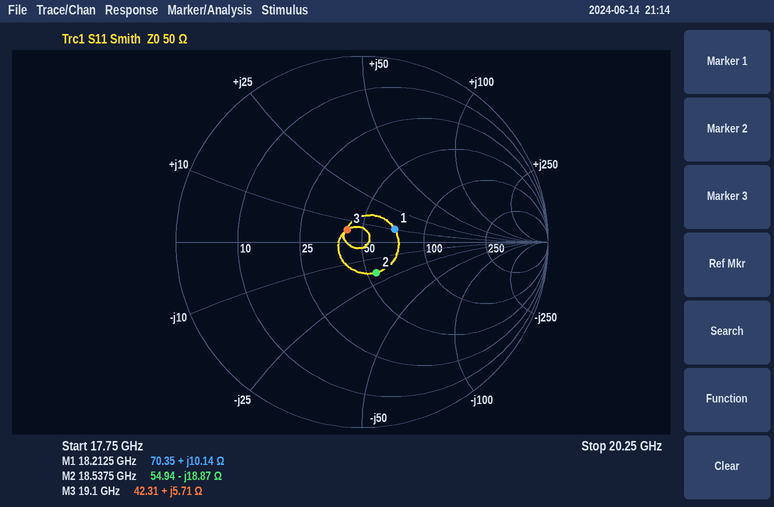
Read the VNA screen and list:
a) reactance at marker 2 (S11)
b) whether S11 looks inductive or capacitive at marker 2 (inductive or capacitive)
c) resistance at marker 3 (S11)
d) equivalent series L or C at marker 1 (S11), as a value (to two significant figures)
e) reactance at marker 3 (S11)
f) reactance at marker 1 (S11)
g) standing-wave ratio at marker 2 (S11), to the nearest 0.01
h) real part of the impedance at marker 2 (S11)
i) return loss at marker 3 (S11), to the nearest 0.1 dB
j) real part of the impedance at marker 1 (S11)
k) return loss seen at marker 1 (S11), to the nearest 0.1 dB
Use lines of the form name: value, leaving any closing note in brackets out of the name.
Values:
reactance at marker 2: -18.87 Ω
whether S11 looks inductive or capacitive at marker 2: capacitive
resistance at marker 3: 42.31 Ω
equivalent series L or C at marker 1 (S11), as a value: 89 pH
reactance at marker 3: +5.71 Ω
reactance at marker 1: +10.14 Ω
standing-wave ratio at marker 2 (S11), to the nearest 0.01: 1.45
real part of the impedance at marker 2: 54.94 Ω
return loss at marker 3 (S11), to the nearest 0.1 dB: 19.7 dB
real part of the impedance at marker 1: 70.35 Ω
return loss seen at marker 1 (S11), to the nearest 0.1 dB: 14.5 dB
